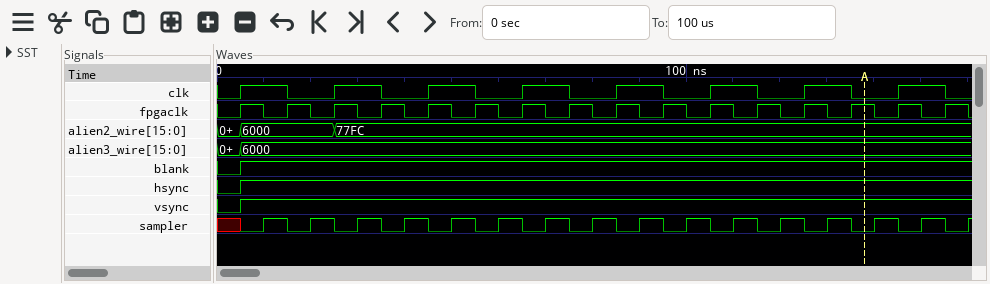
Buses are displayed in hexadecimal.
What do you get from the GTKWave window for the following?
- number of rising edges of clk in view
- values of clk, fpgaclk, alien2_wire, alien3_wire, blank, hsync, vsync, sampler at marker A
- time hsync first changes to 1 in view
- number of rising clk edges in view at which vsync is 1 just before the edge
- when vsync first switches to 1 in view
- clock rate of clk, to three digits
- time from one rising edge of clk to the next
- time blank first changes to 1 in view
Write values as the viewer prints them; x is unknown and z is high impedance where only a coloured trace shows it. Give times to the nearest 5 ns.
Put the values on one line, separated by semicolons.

8; clk=0, fpgaclk=1, alien2_wire=77FC, alien3_wire=6000, blank=1, hsync=1, vsync=1, sampler=0; 5 ns; 7; 5 ns; 50.0 MHz; 20 ns; 5 ns
